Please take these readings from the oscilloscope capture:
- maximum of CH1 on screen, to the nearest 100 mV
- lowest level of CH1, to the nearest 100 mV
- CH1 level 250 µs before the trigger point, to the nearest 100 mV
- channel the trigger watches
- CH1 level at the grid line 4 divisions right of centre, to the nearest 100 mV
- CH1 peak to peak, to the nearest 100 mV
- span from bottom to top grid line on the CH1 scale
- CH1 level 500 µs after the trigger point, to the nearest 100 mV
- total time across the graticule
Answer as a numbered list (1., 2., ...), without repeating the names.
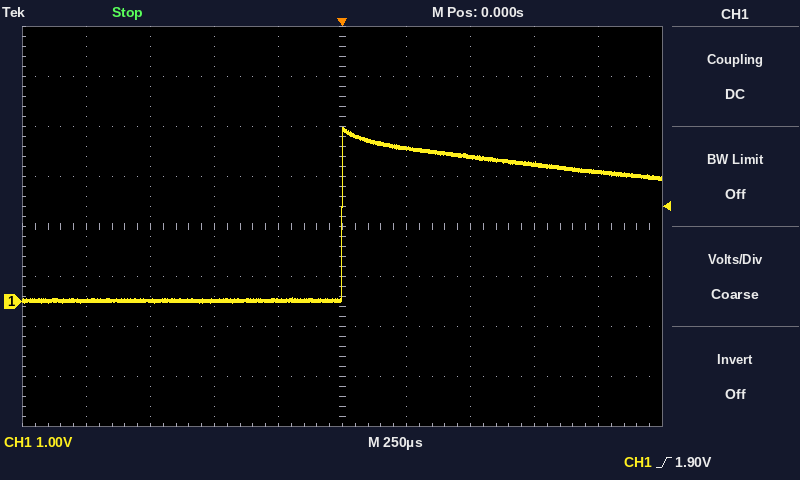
1. 3.5 V
2. 0.0 V
3. 0.0 V
4. CH1
5. 2.6 V
6. 3.5 V
7. 8 V
8. 2.9 V
9. 2.5 ms
